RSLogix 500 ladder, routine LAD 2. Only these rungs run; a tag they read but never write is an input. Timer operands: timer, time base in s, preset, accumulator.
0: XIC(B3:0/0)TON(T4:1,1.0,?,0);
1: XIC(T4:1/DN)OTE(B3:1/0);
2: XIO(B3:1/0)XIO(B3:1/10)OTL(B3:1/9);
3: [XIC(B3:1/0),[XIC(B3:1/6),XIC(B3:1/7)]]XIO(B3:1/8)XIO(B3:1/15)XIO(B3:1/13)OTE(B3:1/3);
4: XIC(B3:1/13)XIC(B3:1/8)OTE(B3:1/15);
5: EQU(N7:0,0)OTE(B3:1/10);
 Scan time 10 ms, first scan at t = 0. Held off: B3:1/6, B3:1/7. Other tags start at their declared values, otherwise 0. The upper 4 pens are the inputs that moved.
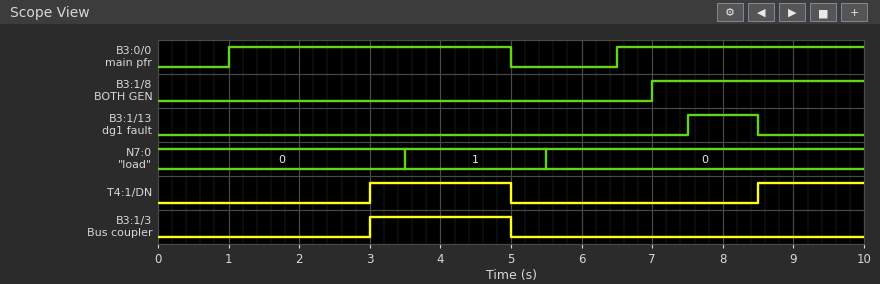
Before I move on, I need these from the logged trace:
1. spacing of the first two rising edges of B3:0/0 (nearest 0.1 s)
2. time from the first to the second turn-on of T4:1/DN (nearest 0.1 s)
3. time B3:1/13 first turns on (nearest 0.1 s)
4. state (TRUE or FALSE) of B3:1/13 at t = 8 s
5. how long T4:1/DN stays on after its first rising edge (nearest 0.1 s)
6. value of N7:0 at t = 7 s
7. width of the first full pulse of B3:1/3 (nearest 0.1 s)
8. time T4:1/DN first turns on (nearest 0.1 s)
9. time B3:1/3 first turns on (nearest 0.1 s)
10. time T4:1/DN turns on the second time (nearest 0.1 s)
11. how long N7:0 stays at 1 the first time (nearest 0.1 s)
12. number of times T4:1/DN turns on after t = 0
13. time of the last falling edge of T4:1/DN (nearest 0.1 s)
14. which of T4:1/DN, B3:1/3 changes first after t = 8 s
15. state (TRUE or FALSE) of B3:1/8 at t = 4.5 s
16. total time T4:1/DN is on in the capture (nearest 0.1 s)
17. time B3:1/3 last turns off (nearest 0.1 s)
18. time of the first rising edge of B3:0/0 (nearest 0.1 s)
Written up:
5.5 s
5.5 s
7.5 s
TRUE
2.0 s
0
2.0 s
3.0 s
3.0 s
8.5 s
2.0 s
2
5.0 s
T4:1/DN
FALSE
3.5 s
5.0 s
1.0 s
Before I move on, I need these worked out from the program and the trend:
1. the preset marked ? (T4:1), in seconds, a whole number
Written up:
2 s
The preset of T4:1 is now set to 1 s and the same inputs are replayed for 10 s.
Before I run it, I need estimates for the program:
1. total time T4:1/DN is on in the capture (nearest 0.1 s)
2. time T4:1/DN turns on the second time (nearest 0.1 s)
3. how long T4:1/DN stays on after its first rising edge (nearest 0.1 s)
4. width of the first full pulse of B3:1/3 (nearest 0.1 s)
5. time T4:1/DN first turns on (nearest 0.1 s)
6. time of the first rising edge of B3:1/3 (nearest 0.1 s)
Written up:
5.5 s
7.5 s
3.0 s
3.0 s
2.0 s
2.0 s
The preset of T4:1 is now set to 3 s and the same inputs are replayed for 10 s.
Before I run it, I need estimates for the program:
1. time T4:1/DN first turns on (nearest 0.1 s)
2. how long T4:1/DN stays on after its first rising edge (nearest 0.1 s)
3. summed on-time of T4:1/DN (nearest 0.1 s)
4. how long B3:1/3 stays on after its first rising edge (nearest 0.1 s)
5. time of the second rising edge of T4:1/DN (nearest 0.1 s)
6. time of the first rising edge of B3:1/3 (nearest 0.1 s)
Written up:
4.0 s
1.0 s
1.5 s
1.0 s
9.5 s
4.0 s
